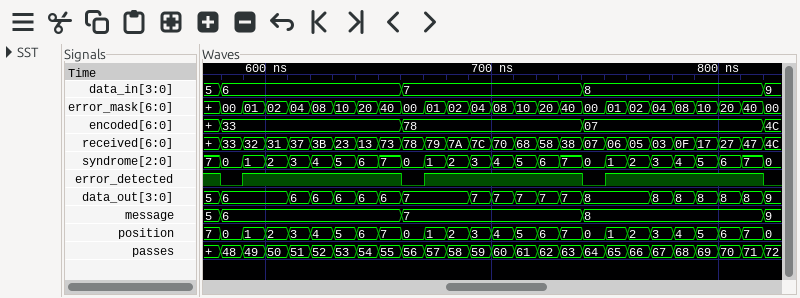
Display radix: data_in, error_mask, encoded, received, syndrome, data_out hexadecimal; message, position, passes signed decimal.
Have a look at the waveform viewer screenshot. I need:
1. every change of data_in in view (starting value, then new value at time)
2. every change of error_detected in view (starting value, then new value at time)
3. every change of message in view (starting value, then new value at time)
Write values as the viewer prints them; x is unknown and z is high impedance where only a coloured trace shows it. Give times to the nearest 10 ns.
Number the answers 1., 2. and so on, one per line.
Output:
1. 5, 6 at 580 ns, 7 at 660 ns, 8 at 740 ns, 9 at 820 ns
2. 1, 0 at 580 ns, 1 at 590 ns, 0 at 660 ns, 1 at 670 ns, 0 at 740 ns, 1 at 750 ns, 0 at 820 ns
3. 5, 6 at 580 ns, 7 at 660 ns, 8 at 740 ns, 9 at 820 ns
